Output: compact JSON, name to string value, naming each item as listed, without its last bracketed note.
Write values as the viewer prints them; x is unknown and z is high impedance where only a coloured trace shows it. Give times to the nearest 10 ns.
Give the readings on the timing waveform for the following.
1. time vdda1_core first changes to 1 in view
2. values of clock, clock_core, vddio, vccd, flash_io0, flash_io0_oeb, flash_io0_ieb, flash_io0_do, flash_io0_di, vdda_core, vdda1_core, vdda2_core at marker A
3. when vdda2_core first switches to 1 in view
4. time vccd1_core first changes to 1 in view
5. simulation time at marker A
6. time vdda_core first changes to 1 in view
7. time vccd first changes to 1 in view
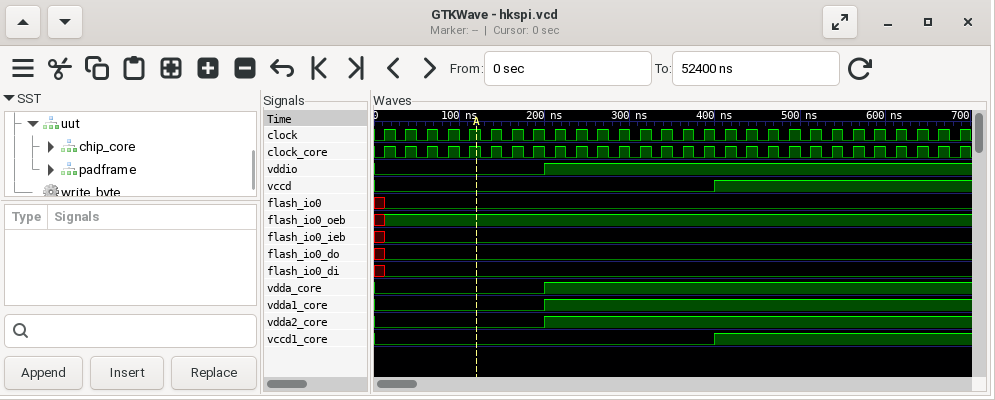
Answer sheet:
{"time vdda1_core first changes to 1 in view": "200 ns", "values of clock, clock_core, vddio, vccd, flash_io0, flash_io0_oeb, flash_io0_ieb, flash_io0_do, flash_io0_di, vdda_core, vdda1_core, vdda2_core at marker A": "clock=1, clock_core=1, vddio=0, vccd=0, flash_io0=0, flash_io0_oeb=1, flash_io0_ieb=0, flash_io0_do=0, flash_io0_di=0, vdda_core=0, vdda1_core=0, vdda2_core=0", "when vdda2_core first switches to 1 in view": "200 ns", "time vccd1_core first changes to 1 in view": "400 ns", "simulation time at marker A": "120 ns", "time vdda_core first changes to 1 in view": "200 ns", "time vccd first changes to 1 in view": "400 ns"}
